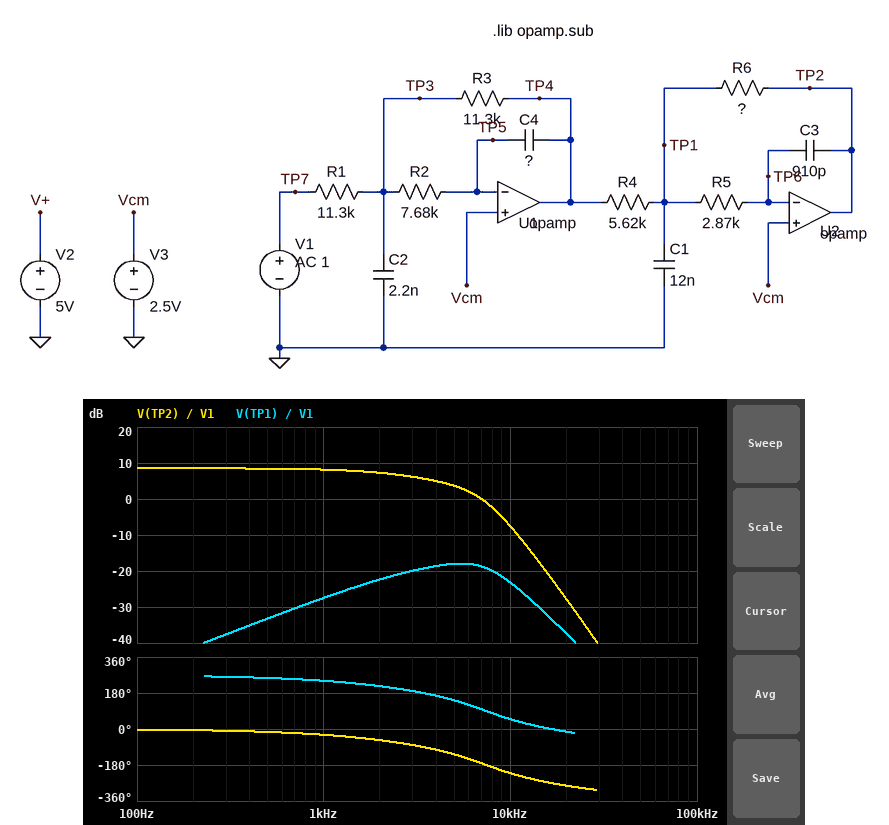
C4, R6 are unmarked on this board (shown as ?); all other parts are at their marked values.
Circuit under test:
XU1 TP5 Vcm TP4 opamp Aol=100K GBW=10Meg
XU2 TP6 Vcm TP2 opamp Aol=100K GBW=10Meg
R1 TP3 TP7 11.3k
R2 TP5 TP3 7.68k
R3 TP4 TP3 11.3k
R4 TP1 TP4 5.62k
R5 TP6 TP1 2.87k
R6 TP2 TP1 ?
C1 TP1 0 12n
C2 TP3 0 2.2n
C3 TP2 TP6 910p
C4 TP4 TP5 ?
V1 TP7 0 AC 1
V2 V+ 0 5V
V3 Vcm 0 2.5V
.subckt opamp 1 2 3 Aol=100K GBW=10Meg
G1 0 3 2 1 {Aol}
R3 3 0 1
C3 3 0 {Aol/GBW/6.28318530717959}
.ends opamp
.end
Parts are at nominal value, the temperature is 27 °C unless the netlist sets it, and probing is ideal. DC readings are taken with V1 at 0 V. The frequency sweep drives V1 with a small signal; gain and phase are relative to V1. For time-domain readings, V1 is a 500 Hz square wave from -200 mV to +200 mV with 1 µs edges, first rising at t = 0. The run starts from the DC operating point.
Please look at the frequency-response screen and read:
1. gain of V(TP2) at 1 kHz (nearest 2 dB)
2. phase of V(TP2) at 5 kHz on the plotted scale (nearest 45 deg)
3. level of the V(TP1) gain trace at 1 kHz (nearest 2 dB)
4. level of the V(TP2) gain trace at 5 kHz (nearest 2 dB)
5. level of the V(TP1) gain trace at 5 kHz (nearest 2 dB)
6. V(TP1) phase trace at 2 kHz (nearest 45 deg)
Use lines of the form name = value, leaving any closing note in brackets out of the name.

gain of V(TP2) at 1 kHz = 8 dB
phase of V(TP2) at 5 kHz on the plotted scale = -135 deg
level of the V(TP1) gain trace at 1 kHz = -28 dB
level of the V(TP2) gain trace at 5 kHz = 4 dB
level of the V(TP1) gain trace at 5 kHz = -18 dB
V(TP1) phase trace at 2 kHz = 225 deg
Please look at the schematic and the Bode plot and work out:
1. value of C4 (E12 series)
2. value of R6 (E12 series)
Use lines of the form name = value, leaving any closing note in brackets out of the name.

value of C4 = 2.2 nF
value of R6 = 15 kΩ
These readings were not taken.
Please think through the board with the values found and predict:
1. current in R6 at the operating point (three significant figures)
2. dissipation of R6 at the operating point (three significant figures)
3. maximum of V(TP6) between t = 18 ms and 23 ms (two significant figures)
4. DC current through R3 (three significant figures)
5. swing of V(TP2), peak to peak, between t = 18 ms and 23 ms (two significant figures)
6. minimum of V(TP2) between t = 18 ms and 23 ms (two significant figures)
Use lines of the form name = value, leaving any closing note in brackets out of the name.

current in R6 at the operating point = 445 µA
dissipation of R6 at the operating point = 2.97 mW
maximum of V(TP6) between t = 18 ms and 23 ms = 2.5 V
DC current through R3 = 221 µA
swing of V(TP2), peak to peak, between t = 18 ms and 23 ms = 1.1 V
minimum of V(TP2) between t = 18 ms and 23 ms = -4.7 V
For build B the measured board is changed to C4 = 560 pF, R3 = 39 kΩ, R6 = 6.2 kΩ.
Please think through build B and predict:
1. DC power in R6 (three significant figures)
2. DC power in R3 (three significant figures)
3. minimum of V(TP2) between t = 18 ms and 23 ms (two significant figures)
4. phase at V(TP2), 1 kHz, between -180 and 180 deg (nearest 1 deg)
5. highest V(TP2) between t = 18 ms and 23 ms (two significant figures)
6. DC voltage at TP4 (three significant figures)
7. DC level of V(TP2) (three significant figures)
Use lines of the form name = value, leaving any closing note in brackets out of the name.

DC power in R6 = 14.6 mW
DC power in R3 = 1.91 mW
minimum of V(TP2) between t = 18 ms and 23 ms = -7.8 V
phase at V(TP2), 1 kHz, between -180 and 180 deg = -19 deg
highest V(TP2) between t = 18 ms and 23 ms = -6.3 V
DC voltage at TP4 = 11.1 V
DC level of V(TP2) = -7.02 V
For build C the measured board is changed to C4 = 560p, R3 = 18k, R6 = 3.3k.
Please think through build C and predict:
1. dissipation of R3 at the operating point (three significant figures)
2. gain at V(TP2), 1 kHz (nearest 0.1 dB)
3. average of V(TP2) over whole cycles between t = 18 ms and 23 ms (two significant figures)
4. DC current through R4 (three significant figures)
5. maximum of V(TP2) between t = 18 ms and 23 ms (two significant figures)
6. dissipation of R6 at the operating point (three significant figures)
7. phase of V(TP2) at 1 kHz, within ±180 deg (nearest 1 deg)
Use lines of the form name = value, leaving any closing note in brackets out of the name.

dissipation of R3 at the operating point = 881 µW
gain at V(TP2), 1 kHz = -0.6 dB
average of V(TP2) over whole cycles between t = 18 ms and 23 ms = 160 mV
DC current through R4 = 709 µA
maximum of V(TP2) between t = 18 ms and 23 ms = 400 mV
dissipation of R6 at the operating point = 1.66 mW
phase of V(TP2) at 1 kHz, within ±180 deg = -10 deg
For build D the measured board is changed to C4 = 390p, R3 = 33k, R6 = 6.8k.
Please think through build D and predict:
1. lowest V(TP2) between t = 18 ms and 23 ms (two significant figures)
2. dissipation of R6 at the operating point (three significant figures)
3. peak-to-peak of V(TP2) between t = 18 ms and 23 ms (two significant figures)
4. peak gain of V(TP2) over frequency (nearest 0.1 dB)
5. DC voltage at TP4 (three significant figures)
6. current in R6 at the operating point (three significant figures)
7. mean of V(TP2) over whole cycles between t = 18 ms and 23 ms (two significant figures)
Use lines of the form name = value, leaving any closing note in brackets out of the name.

lowest V(TP2) between t = 18 ms and 23 ms = -7.2 V
dissipation of R6 at the operating point = 11.5 mW
peak-to-peak of V(TP2) between t = 18 ms and 23 ms = 1.8 V
peak gain of V(TP2) over frequency = 11.3 dB
DC voltage at TP4 = 9.80 V
current in R6 at the operating point = 1.30 mA
mean of V(TP2) over whole cycles between t = 18 ms and 23 ms = -6.3 V
